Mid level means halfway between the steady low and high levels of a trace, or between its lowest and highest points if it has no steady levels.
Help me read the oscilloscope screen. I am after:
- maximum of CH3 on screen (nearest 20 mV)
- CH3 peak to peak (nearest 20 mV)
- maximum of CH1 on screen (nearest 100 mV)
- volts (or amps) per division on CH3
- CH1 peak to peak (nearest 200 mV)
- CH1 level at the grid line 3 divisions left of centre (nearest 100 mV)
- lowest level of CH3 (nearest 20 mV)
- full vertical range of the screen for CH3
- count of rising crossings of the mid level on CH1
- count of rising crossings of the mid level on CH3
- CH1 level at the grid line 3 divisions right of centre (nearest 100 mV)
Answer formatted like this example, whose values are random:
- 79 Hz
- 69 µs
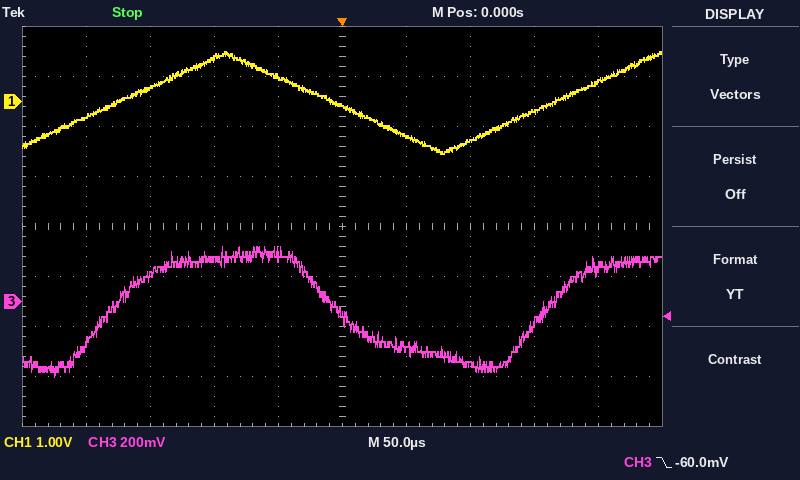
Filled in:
- 220 mV
- 520 mV
- 1.0 V
- 200 mV
- 2.0 V
- 300 mV
- -300 mV
- 1.6 V
- 2
- 2
- -200 mV
